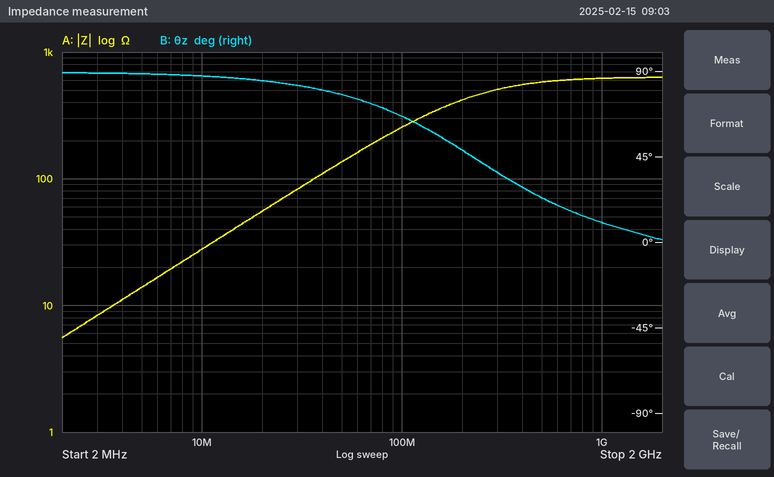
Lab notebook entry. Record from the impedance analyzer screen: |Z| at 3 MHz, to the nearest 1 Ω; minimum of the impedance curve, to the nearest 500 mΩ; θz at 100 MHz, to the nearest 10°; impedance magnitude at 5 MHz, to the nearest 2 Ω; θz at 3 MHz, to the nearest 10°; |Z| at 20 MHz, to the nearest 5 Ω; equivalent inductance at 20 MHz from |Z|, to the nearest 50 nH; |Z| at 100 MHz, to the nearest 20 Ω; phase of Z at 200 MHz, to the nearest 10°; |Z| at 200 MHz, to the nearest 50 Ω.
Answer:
8 Ω
5.5 Ω
70°
14 Ω
90°
55 Ω
450 nH
260 Ω
50°
400 Ω
